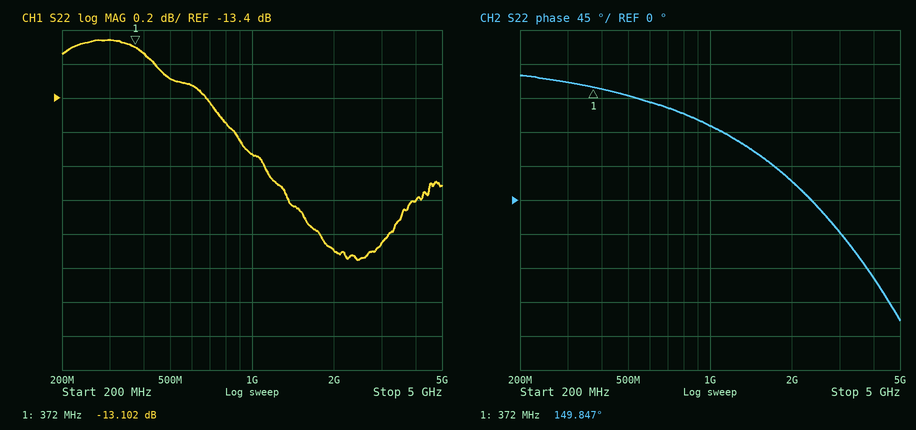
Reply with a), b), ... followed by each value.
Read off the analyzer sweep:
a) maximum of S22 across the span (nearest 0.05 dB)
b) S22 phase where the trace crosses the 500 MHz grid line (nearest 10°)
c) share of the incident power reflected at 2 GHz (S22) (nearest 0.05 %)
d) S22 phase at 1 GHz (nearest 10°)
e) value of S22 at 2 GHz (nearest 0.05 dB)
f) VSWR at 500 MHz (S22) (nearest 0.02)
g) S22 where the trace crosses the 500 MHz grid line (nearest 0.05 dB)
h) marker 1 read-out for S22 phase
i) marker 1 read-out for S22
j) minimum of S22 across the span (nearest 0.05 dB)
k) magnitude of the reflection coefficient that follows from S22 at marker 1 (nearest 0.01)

a) -13.05 dB
b) 140°
c) 3.70 %
d) 100°
e) -14.30 dB
f) 1.56
g) -13.30 dB
h) 149.847°
i) -13.102 dB
j) -14.35 dB
k) 0.22
